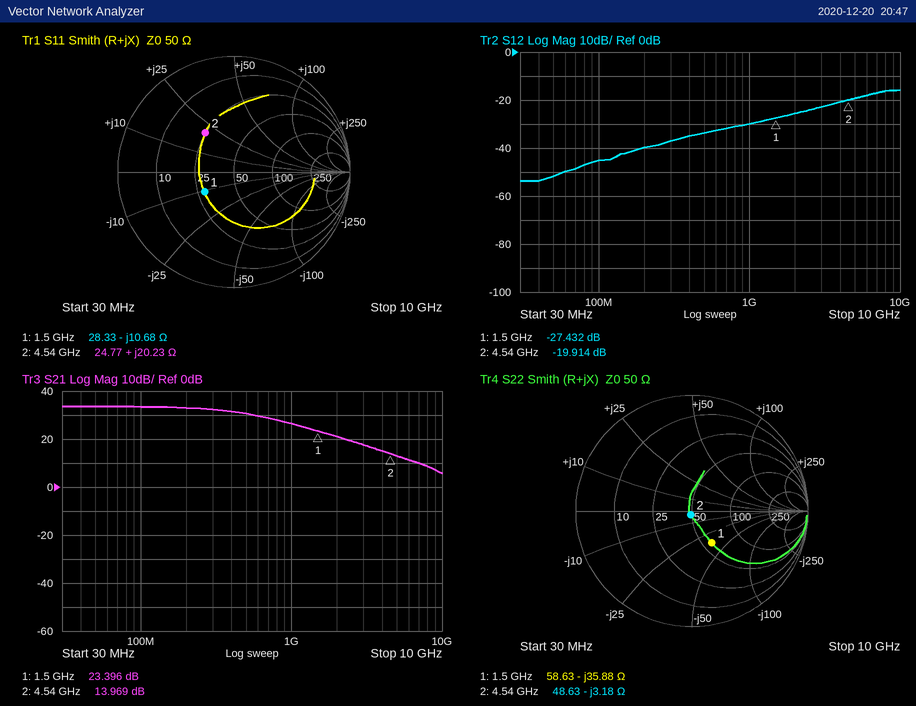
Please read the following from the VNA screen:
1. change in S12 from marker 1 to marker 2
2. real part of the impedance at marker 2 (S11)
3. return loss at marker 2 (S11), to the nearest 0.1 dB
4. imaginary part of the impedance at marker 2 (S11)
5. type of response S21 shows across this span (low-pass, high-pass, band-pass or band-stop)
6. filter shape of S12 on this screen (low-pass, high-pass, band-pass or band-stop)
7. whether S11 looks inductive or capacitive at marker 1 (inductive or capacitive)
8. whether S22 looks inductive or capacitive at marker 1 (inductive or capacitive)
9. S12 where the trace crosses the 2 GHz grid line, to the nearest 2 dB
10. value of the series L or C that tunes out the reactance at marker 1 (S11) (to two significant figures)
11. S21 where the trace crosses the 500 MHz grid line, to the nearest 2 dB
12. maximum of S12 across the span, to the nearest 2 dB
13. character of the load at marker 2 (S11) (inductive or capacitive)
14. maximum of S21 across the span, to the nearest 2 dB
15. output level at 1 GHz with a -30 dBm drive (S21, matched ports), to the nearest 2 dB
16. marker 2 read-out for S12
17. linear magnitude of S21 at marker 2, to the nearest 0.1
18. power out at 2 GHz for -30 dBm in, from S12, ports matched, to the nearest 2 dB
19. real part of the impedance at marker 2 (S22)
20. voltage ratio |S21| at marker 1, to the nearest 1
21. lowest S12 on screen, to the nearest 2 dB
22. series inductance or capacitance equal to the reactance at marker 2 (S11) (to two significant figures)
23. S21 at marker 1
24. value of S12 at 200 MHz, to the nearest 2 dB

7.518 dB
24.77 Ω
7.6 dB
+20.23 Ω
low-pass
high-pass
capacitive
capacitive
-26 dB
1.1 nH
30 dB
-16 dB
inductive
34 dB
-4 dBm
-19.914 dB
5.0
-56 dBm
48.63 Ω
15
-54 dB
710 pH
23.396 dB
-40 dB
